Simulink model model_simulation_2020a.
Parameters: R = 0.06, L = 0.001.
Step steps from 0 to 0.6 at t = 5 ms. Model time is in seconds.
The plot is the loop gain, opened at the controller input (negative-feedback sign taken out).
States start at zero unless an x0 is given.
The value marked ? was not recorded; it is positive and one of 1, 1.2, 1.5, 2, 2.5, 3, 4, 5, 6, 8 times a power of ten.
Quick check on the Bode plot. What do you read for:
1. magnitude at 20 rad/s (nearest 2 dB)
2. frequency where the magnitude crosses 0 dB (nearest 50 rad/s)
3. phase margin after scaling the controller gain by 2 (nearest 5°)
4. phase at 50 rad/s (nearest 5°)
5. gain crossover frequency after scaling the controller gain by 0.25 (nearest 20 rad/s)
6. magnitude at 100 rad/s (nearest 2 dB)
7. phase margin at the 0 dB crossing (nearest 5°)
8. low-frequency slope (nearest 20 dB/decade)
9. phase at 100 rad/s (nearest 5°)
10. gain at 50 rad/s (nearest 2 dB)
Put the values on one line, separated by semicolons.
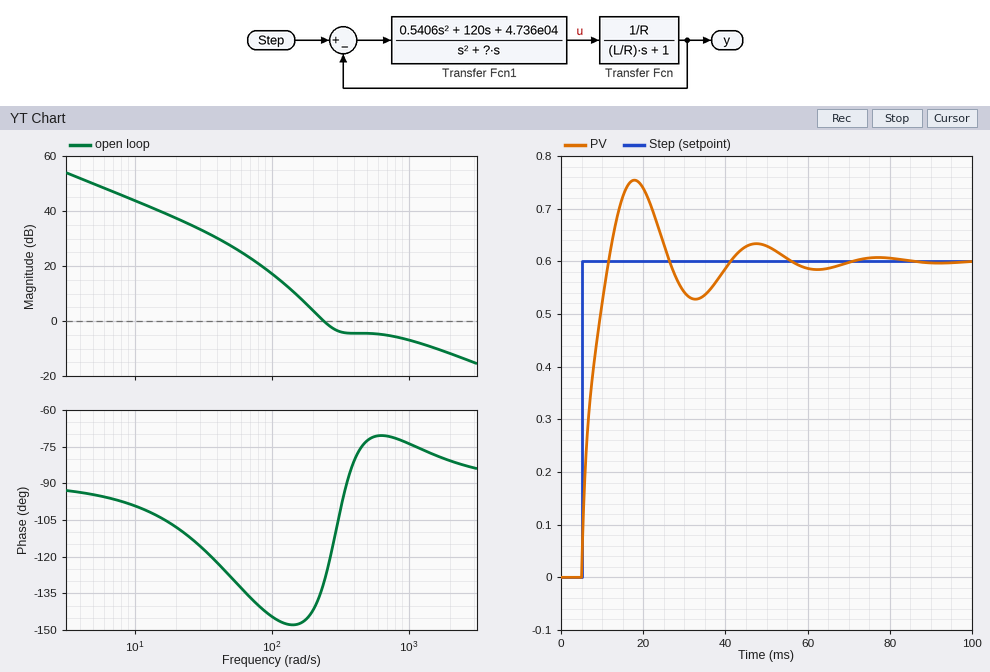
38 dB; 250 rad/s; 110°; -130°; 140 rad/s; 18 dB; 50°; -20 dB/decade; -145°; 28 dB
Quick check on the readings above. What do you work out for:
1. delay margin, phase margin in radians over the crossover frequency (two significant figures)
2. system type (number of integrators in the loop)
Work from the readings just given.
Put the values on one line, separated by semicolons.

0.0035 s; 1
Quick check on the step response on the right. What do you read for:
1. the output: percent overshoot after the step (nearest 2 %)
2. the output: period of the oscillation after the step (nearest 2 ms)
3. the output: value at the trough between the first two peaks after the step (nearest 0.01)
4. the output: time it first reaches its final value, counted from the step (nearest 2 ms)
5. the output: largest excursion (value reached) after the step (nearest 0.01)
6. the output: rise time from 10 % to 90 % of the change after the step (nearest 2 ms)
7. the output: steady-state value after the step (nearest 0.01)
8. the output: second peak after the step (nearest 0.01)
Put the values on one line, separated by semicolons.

26 %; 30 ms; 0.53; 6 ms; 0.75; 6 ms; 0.60; 0.63
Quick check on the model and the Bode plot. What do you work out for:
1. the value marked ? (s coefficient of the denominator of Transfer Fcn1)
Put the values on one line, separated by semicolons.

500
